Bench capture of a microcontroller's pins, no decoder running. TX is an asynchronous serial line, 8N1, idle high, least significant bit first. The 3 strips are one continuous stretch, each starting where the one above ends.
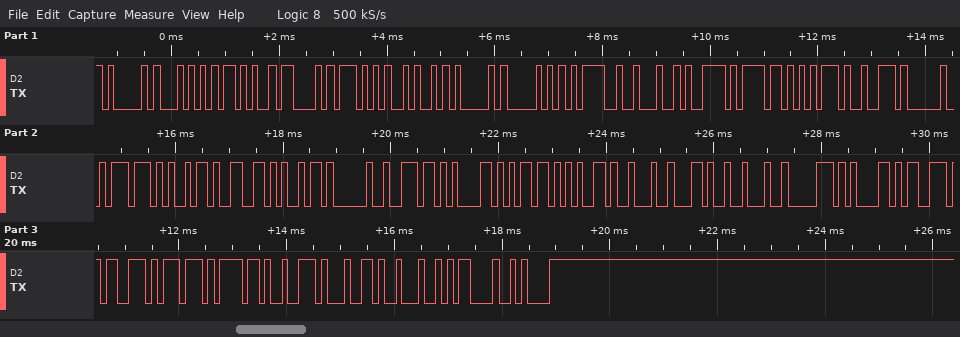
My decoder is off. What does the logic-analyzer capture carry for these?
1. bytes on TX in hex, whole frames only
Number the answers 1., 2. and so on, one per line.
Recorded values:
1. 41 54 2B 43 57 4A 41 50 3D 22 79 6F 75 72 20 77 69 66 69 20 6E 61 6D 65 22 2C 22 70 61 73 73 77 6F 72 64 22 0D 0A
